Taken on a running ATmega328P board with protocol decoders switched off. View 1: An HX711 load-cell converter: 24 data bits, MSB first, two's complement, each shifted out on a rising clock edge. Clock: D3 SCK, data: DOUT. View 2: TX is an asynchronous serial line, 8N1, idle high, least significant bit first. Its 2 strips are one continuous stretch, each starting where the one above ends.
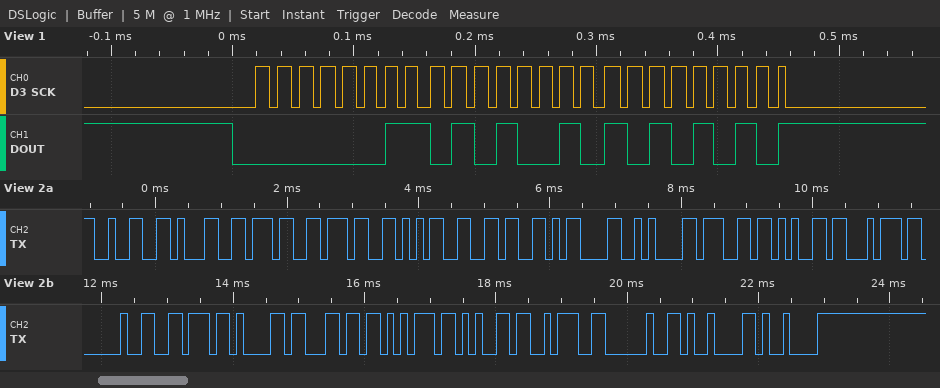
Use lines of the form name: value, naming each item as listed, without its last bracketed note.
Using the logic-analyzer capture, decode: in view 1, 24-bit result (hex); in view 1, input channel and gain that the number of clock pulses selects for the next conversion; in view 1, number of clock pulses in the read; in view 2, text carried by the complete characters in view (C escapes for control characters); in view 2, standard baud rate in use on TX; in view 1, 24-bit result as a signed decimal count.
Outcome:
in view 1, 24-bit result: 0x0352AA
in view 1, input channel and gain that the number of clock pulses selects for the next conversion: channel A, gain 128
in view 1, number of clock pulses in the read: 25
in view 2, text carried by the complete characters in view: "217756\r\nget value: \t\t"
in view 2, standard baud rate in use on TX: 9600 baud
in view 1, 24-bit result as a signed decimal count: 217770
